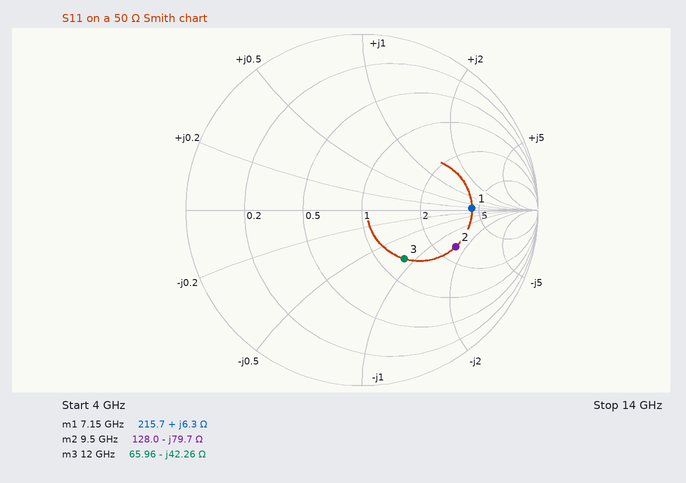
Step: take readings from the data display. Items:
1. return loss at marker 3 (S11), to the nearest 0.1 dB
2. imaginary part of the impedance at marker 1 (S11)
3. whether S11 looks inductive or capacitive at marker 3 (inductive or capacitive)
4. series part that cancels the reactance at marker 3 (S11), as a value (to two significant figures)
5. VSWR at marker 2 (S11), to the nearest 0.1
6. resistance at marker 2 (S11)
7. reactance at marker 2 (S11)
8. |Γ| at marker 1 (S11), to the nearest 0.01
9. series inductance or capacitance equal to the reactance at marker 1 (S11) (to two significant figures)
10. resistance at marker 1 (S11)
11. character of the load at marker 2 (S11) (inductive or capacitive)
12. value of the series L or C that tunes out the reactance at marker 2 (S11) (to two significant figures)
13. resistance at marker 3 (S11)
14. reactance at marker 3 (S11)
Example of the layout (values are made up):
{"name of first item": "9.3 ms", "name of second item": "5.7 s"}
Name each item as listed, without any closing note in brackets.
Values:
{"return loss at marker 3 (S11), to the nearest 0.1 dB": "8.7 dB", "imaginary part of the impedance at marker 1": "+6.3 Ω", "whether S11 looks inductive or capacitive at marker 3": "capacitive", "series part that cancels the reactance at marker 3 (S11), as a value": "560 pH", "VSWR at marker 2 (S11), to the nearest 0.1": "3.7", "resistance at marker 2": "128.0 Ω", "reactance at marker 2": "-79.7 Ω", "|Γ| at marker 1 (S11), to the nearest 0.01": "0.62", "series inductance or capacitance equal to the reactance at marker 1 (S11)": "140 pH", "resistance at marker 1": "215.7 Ω", "character of the load at marker 2 (S11)": "capacitive", "value of the series L or C that tunes out the reactance at marker 2 (S11)": "1.3 nH", "resistance at marker 3": "65.96 Ω", "reactance at marker 3": "-42.26 Ω"}
